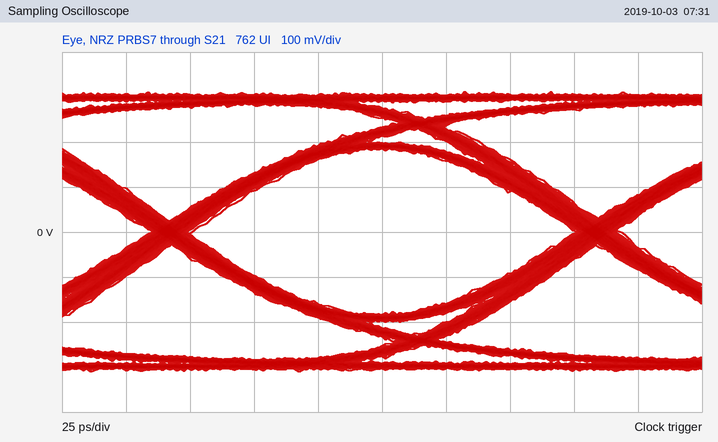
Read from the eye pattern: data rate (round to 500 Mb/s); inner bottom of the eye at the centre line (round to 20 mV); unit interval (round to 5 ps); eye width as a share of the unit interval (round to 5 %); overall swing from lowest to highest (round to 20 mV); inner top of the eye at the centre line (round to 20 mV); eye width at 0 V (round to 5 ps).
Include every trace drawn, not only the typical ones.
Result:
6.0 Gb/s
-180 mV
165 ps
90 %
620 mV
180 mV
150 ps
